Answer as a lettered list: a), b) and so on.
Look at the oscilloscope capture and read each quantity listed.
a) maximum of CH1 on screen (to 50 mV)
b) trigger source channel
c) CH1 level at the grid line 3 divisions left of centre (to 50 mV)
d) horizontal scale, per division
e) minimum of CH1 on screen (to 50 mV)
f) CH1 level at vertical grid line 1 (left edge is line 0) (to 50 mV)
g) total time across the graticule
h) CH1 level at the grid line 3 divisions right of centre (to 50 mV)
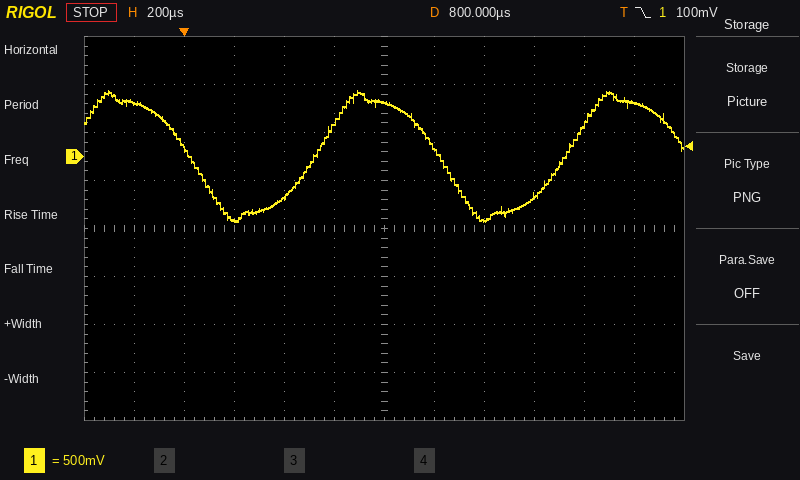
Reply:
a) 700 mV
b) CH1
c) -650 mV
d) 200 µs
e) -700 mV
f) 550 mV
g) 2.4 ms
h) -400 mV
